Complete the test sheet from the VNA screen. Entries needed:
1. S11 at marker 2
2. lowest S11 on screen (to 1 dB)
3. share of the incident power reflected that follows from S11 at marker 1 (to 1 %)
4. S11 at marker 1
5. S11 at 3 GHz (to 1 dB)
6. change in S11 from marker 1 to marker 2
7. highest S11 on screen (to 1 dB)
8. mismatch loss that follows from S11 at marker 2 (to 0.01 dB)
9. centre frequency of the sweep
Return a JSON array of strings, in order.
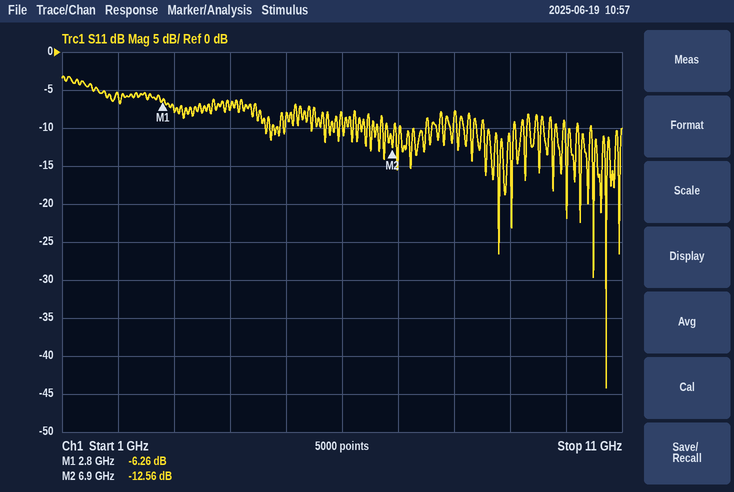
["-12.56 dB", "-44 dB", "24 %", "-6.26 dB", "-8 dB", "-6.30 dB", "-3 dB", "0.25 dB", "6 GHz"]
